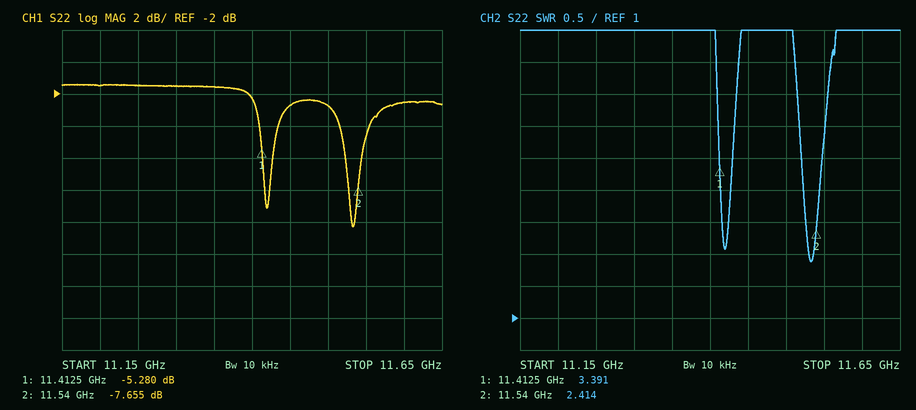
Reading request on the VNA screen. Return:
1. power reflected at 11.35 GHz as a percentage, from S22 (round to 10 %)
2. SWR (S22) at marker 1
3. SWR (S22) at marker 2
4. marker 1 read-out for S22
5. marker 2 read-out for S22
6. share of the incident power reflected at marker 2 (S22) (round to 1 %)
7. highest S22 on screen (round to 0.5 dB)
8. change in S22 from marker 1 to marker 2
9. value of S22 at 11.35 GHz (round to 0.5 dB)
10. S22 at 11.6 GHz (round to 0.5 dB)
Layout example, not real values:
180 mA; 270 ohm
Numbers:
70 %; 3.391; 2.414; -5.280 dB; -7.655 dB; 17 %; -1.5 dB; -2.375 dB; -1.5 dB; -2.5 dB
